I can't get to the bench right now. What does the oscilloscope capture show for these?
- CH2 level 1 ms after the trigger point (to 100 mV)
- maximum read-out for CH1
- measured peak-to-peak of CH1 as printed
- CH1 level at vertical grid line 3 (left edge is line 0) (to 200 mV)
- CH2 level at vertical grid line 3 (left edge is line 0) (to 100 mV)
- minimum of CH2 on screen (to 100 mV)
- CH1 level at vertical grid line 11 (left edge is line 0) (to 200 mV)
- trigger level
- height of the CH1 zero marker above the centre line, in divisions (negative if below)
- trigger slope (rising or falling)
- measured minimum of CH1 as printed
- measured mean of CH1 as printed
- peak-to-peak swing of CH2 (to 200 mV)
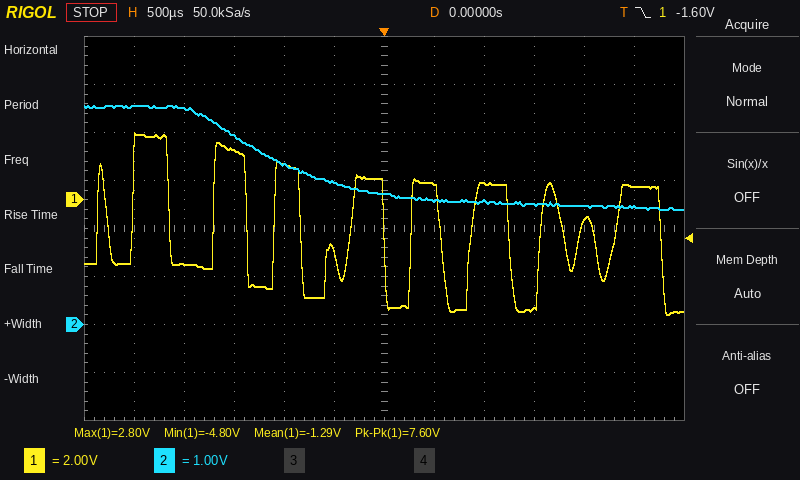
2.6 V
2.80 V
7.60 V
2.0 V
3.9 V
2.4 V
600 mV
-1.60 V
+0.6 div
falling
-4.80 V
-1.29 V
2.2 V
